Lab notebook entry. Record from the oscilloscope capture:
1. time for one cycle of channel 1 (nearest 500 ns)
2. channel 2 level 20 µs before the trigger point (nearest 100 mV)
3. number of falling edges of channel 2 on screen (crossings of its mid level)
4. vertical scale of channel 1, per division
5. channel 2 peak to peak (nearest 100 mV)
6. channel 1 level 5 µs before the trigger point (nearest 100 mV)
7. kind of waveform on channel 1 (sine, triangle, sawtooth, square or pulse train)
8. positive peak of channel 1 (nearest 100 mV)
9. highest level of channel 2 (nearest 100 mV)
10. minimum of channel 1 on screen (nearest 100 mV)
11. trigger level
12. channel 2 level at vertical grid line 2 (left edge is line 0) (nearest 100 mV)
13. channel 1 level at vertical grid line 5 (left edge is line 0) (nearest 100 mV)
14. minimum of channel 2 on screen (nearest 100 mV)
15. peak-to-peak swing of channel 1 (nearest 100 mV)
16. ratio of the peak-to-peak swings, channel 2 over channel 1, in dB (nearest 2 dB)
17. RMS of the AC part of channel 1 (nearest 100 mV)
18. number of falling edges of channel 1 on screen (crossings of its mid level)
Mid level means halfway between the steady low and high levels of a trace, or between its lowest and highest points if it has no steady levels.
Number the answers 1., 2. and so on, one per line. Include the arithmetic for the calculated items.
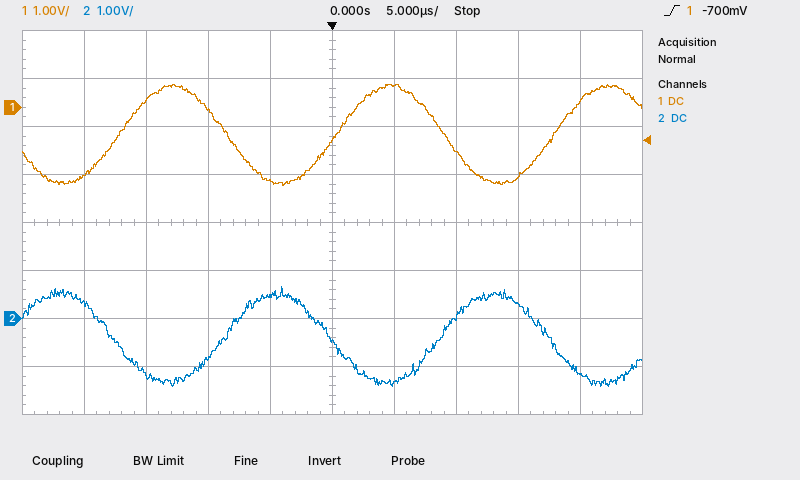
1. 17.5 µs
2. 300 mV
3. 3
4. 1 V
5. 700 mV − (-1.4 V) = 2.1 V
6. -1.5 V
7. sine
8. 500 mV
9. 700 mV
10. -1.6 V
11. -700 mV
12. -1.2 V
13. -700 mV
14. -1.4 V
15. 500 mV − (-1.6 V) = 2.1 V
16. 20 log10(2.1 V / 2.1 V) ≈ 0 dB
17. 2.1 V / (2√2) ≈ 742 mV, so 700 mV to the nearest 100 mV
18. 2
